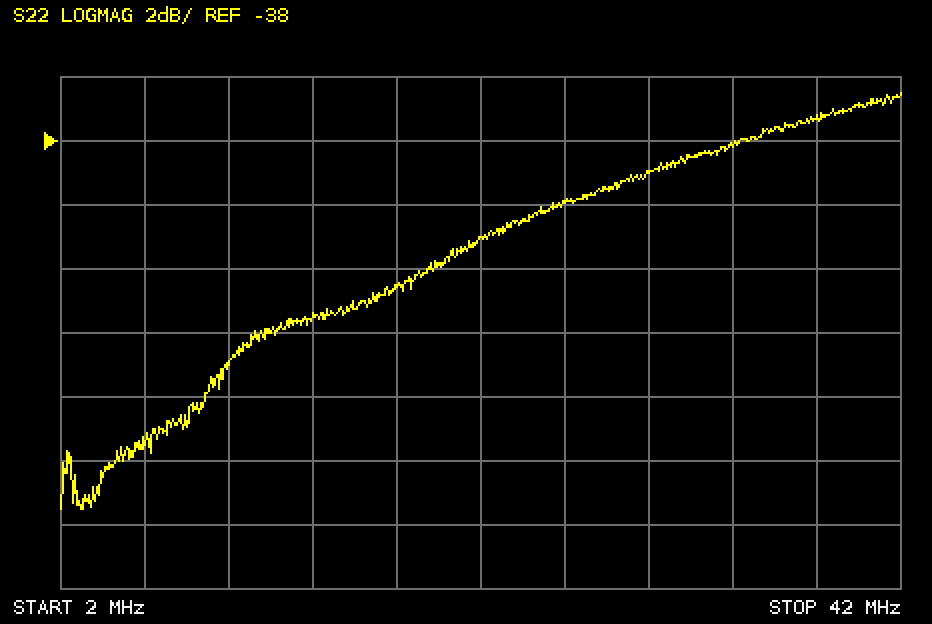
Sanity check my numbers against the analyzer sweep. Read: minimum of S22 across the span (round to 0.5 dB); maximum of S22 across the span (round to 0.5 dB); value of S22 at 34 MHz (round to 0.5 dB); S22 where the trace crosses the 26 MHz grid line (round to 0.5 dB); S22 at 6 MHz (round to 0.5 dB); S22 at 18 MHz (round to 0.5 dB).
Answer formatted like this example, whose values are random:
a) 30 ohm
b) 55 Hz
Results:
a) -49.5 dB
b) -36.5 dB
c) -38.0 dB
d) -40.0 dB
e) -47.5 dB
f) -42.5 dB
